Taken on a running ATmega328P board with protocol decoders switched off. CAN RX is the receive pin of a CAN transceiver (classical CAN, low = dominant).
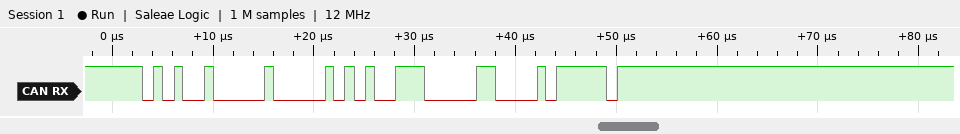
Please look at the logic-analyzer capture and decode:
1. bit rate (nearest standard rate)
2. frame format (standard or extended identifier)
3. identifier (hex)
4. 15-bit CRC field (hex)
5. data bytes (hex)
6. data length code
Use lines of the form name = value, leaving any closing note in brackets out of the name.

bit rate = 1000 kbit/s
frame format = standard
identifier = 0x520
15-bit CRC field = 0x042F
data bytes = 4E
data length code = 1
